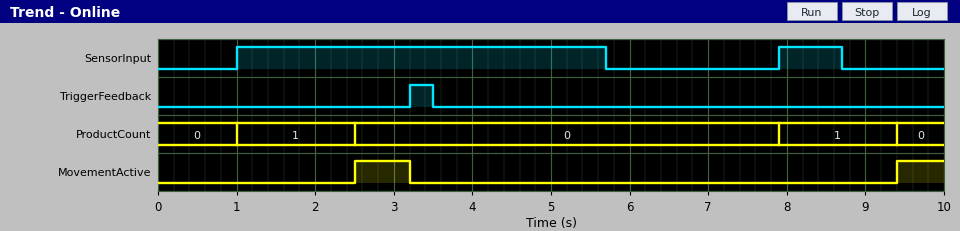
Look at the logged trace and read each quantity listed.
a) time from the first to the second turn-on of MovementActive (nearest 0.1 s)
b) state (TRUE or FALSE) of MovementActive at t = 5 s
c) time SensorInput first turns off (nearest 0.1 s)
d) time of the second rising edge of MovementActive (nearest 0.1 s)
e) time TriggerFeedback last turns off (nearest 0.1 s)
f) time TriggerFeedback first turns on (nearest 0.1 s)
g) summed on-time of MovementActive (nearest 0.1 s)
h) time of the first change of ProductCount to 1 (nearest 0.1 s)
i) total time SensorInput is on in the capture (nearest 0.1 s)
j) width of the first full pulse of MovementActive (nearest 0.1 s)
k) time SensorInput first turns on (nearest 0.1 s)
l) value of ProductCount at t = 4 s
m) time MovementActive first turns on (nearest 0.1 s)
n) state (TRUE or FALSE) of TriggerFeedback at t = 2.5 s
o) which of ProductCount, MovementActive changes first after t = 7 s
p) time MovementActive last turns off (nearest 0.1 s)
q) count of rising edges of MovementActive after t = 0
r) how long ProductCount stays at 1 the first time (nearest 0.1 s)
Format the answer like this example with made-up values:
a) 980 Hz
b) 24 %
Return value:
a) 6.9 s
b) FALSE
c) 5.7 s
d) 9.4 s
e) 3.5 s
f) 3.2 s
g) 1.3 s
h) 1.0 s
i) 5.5 s
j) 0.7 s
k) 1.0 s
l) 0
m) 2.5 s
n) FALSE
o) ProductCount
p) 3.2 s
q) 2
r) 1.5 s
